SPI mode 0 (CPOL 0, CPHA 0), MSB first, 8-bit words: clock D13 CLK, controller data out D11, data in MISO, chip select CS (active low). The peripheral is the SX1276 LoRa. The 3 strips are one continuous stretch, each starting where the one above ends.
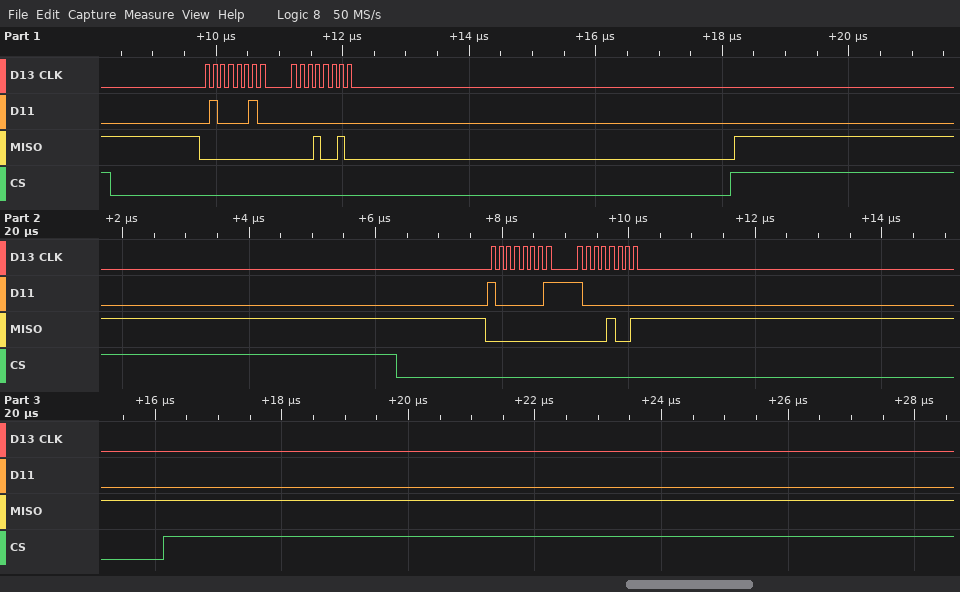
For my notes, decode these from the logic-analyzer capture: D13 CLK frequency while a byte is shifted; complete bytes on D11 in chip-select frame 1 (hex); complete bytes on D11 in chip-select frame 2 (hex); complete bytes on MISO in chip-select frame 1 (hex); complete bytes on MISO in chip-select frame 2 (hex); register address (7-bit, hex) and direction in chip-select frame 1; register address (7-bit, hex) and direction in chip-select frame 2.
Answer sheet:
8 MHz
0x42 0x00
0x81 0x80
0x00 0x12
0x00 0x09
0x42 read
0x01 write
